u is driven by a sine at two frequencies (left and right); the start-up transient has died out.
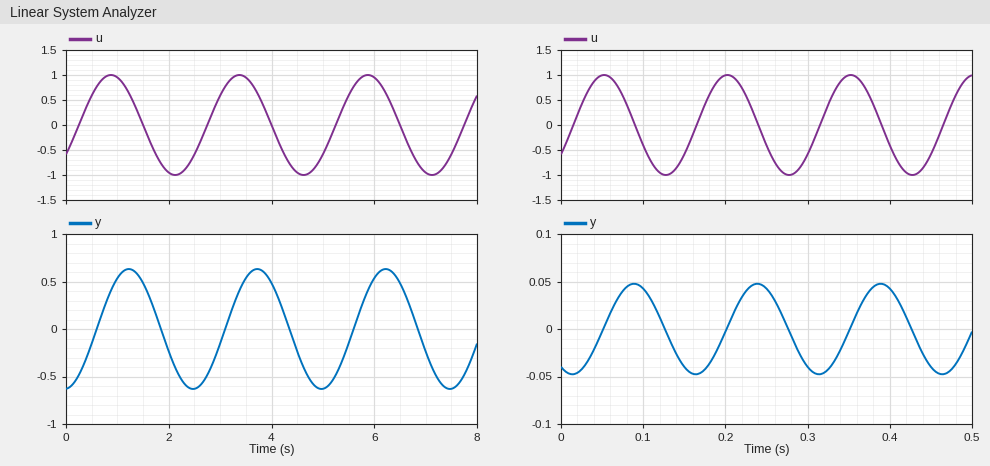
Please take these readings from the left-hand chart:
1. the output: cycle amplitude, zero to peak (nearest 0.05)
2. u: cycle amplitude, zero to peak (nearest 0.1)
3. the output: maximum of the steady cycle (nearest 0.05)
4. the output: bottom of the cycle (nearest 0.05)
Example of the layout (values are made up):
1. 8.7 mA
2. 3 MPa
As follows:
1. 0.65
2. 1.0
3. 0.65
4. -0.65
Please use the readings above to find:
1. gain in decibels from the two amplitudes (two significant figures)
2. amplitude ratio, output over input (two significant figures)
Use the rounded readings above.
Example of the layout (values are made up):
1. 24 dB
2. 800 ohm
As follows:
1. -3.7 dB
2. 0.65
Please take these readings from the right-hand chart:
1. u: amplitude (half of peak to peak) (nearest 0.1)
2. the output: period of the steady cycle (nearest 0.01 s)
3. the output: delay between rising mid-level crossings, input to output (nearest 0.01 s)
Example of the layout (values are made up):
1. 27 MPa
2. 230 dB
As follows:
1. 1.0
2. 0.15 s
3. 0.04 s
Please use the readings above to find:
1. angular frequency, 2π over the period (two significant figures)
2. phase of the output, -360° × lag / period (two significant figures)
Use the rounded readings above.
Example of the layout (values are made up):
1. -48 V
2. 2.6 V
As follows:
1. 42 rad/s
2. -96°
